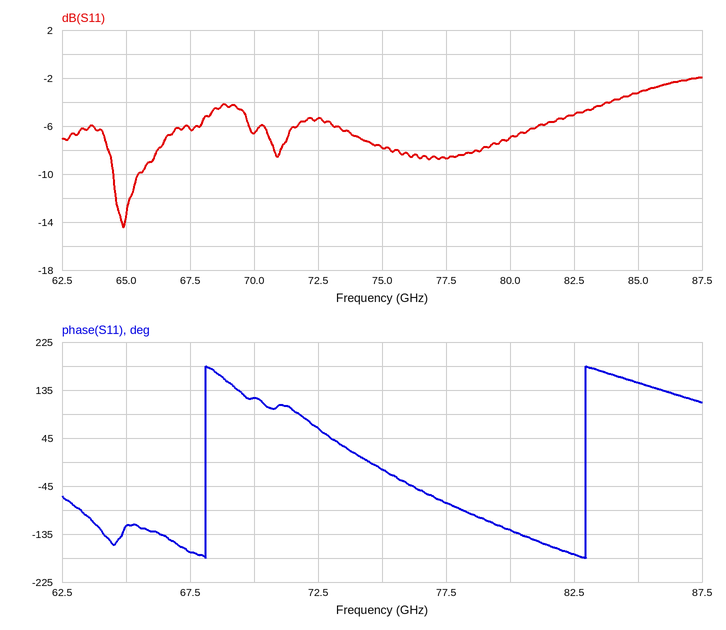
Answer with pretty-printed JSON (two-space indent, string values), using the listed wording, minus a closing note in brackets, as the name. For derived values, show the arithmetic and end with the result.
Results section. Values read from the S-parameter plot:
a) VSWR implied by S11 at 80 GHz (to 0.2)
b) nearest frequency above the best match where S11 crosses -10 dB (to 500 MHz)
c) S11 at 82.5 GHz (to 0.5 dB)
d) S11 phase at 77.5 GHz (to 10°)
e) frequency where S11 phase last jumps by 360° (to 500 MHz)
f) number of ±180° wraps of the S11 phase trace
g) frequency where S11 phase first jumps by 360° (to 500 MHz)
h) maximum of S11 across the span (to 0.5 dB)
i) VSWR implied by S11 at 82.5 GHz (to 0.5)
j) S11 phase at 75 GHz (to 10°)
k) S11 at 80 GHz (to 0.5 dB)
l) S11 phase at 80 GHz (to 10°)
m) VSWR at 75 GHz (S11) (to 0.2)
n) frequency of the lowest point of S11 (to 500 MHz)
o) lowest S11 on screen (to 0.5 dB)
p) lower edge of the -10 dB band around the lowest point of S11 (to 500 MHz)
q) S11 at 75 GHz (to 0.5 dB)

{
  "VSWR implied by S11 at 80 GHz": "|Γ| = 10^(-7/20) = 0.4467; VSWR = (1 + 0.4467)/(1 − 0.4467) ≈ 2.6",
  "nearest frequency above the best match where S11 crosses -10 dB": "65.5 GHz",
  "S11 at 82.5 GHz": "-5.0 dB",
  "S11 phase at 77.5 GHz": "-80°",
  "frequency where S11 phase last jumps by 360°": "83.0 GHz",
  "number of ±180° wraps of the S11 phase trace": "2",
  "frequency where S11 phase first jumps by 360°": "68.0 GHz",
  "maximum of S11 across the span": "-2.0 dB",
  "VSWR implied by S11 at 82.5 GHz": "|Γ| = 10^(-5/20) = 0.5623; VSWR = (1 + 0.5623)/(1 − 0.5623) ≈ 3.57, so 3.5 to the nearest 0.5",
  "S11 phase at 75 GHz": "-10°",
  "S11 at 80 GHz": "-7.0 dB",
  "S11 phase at 80 GHz": "-130°",
  "VSWR at 75 GHz (S11)": "|Γ| = 10^(-8/20) = 0.3981; VSWR = (1 + 0.3981)/(1 − 0.3981) ≈ 2.32, so 2.4 to the nearest 0.2",
  "frequency of the lowest point of S11": "65.0 GHz",
  "lowest S11 on screen": "-14.5 dB",
  "lower edge of the -10 dB band around the lowest point of S11": "64.5 GHz",
  "S11 at 75 GHz": "-8.0 dB"
}
